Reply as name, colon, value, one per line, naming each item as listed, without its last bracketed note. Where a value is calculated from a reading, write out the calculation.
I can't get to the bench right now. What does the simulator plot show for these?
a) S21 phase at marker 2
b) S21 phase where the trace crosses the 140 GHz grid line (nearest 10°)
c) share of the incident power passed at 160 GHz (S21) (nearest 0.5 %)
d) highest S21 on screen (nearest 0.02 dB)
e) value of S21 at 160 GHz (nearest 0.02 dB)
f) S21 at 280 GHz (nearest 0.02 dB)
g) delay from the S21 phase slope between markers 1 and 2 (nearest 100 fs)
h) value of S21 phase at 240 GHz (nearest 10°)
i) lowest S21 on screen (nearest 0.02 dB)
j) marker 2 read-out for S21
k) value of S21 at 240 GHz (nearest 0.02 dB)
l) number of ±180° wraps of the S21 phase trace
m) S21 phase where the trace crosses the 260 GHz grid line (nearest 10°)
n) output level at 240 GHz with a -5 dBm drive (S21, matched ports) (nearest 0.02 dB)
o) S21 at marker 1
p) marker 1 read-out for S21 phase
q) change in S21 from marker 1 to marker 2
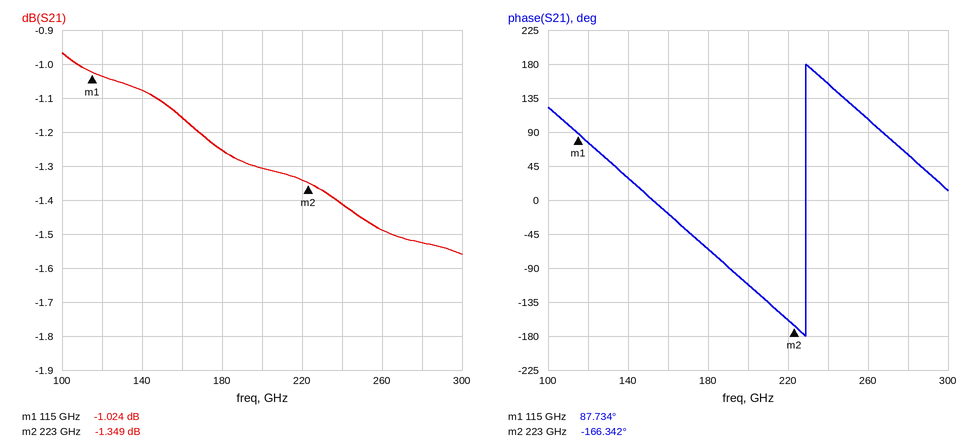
S21 phase at marker 2: -166.342°
S21 phase where the trace crosses the 140 GHz grid line: 30°
share of the incident power passed at 160 GHz (S21): 10^(-1.16/10) ≈ 76.6 %, so 76.5 % to the nearest 0.5 %
highest S21 on screen: -0.96 dB
value of S21 at 160 GHz: -1.16 dB
S21 at 280 GHz: -1.52 dB
delay from the S21 phase slope between markers 1 and 2: −(-166.342° − (87.734°))/(360° × 108 GHz) ≈ 6.5 ps
value of S21 phase at 240 GHz: 150°
lowest S21 on screen: -1.56 dB
marker 2 read-out for S21: -1.349 dB
value of S21 at 240 GHz: -1.42 dB
number of ±180° wraps of the S21 phase trace: 1
S21 phase where the trace crosses the 260 GHz grid line: 110°
output level at 240 GHz with a -5 dBm drive (S21, matched ports): -5 dBm + (-1.42 dB) = -6.42 dBm
S21 at marker 1: -1.024 dB
marker 1 read-out for S21 phase: 87.734°
change in S21 from marker 1 to marker 2: -1.349 − (-1.024) = -0.325 dB
